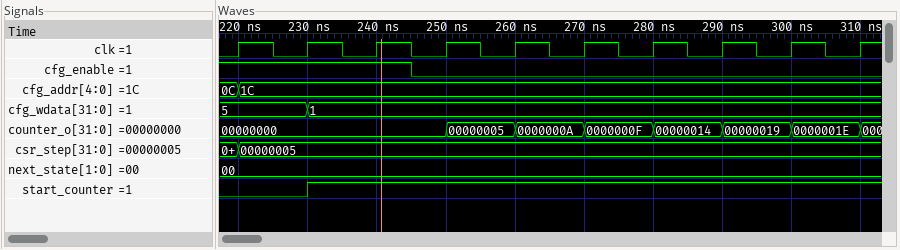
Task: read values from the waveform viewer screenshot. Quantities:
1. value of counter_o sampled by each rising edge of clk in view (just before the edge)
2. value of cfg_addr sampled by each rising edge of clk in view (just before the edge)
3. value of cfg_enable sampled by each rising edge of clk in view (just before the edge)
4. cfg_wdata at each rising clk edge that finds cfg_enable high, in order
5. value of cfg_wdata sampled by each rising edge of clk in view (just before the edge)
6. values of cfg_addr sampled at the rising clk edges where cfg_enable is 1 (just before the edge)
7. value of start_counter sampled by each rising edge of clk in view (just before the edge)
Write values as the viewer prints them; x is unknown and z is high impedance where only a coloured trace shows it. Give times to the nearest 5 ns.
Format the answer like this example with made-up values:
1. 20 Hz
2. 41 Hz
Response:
1. 00000000, 00000000, 00000000, 00000000, 00000005, 0000000A, 0000000F, 00000014, 00000019, 0000001E
2. 0C, 1C, 1C, 1C, 1C, 1C, 1C, 1C, 1C, 1C
3. 1 1 1 0 0 0 0 0 0 0
4. 5, 5, 1
5. 5, 5, 1, 1, 1, 1, 1, 1, 1, 1
6. 0C, 1C, 1C
7. 0 0 1 1 1 1 1 1 1 1
